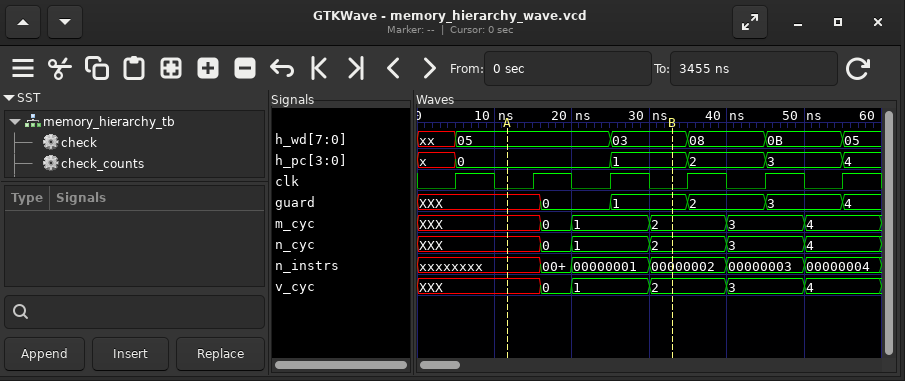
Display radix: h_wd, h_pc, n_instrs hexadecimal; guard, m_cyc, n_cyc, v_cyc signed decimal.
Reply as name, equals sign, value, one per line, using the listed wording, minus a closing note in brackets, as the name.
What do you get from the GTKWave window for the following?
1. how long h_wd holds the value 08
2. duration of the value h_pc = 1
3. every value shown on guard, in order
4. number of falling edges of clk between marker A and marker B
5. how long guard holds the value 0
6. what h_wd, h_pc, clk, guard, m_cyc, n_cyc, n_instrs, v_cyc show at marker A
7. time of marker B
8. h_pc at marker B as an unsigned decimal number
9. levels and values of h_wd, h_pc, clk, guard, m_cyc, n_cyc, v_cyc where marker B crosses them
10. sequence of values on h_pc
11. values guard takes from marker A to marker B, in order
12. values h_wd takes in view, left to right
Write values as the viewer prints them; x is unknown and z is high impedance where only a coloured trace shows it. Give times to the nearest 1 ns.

how long h_wd holds the value 08 = 10 ns
duration of the value h_pc = 1 = 10 ns
every value shown on guard, in order = XXX, 0, 1, 2, 3, 4
number of falling edges of clk between marker A and marker B = 2
how long guard holds the value 0 = 9 ns
what h_wd, h_pc, clk, guard, m_cyc, n_cyc, n_instrs, v_cyc show at marker A = h_wd=05, h_pc=0, clk=0, guard=XXX, m_cyc=XXX, n_cyc=XXX, n_instrs=xxxxxxxx, v_cyc=XXX
time of marker B = 33 ns
h_pc at marker B as an unsigned decimal number = 1
levels and values of h_wd, h_pc, clk, guard, m_cyc, n_cyc, v_cyc where marker B crosses them = h_wd=03, h_pc=1, clk=0, guard=1, m_cyc=2, n_cyc=2, v_cyc=2
sequence of values on h_pc = x, 0, 1, 2, 3, 4
values guard takes from marker A to marker B, in order = XXX, 0, 1
values h_wd takes in view, left to right = xx, 05, 03, 08, 0B, 05
